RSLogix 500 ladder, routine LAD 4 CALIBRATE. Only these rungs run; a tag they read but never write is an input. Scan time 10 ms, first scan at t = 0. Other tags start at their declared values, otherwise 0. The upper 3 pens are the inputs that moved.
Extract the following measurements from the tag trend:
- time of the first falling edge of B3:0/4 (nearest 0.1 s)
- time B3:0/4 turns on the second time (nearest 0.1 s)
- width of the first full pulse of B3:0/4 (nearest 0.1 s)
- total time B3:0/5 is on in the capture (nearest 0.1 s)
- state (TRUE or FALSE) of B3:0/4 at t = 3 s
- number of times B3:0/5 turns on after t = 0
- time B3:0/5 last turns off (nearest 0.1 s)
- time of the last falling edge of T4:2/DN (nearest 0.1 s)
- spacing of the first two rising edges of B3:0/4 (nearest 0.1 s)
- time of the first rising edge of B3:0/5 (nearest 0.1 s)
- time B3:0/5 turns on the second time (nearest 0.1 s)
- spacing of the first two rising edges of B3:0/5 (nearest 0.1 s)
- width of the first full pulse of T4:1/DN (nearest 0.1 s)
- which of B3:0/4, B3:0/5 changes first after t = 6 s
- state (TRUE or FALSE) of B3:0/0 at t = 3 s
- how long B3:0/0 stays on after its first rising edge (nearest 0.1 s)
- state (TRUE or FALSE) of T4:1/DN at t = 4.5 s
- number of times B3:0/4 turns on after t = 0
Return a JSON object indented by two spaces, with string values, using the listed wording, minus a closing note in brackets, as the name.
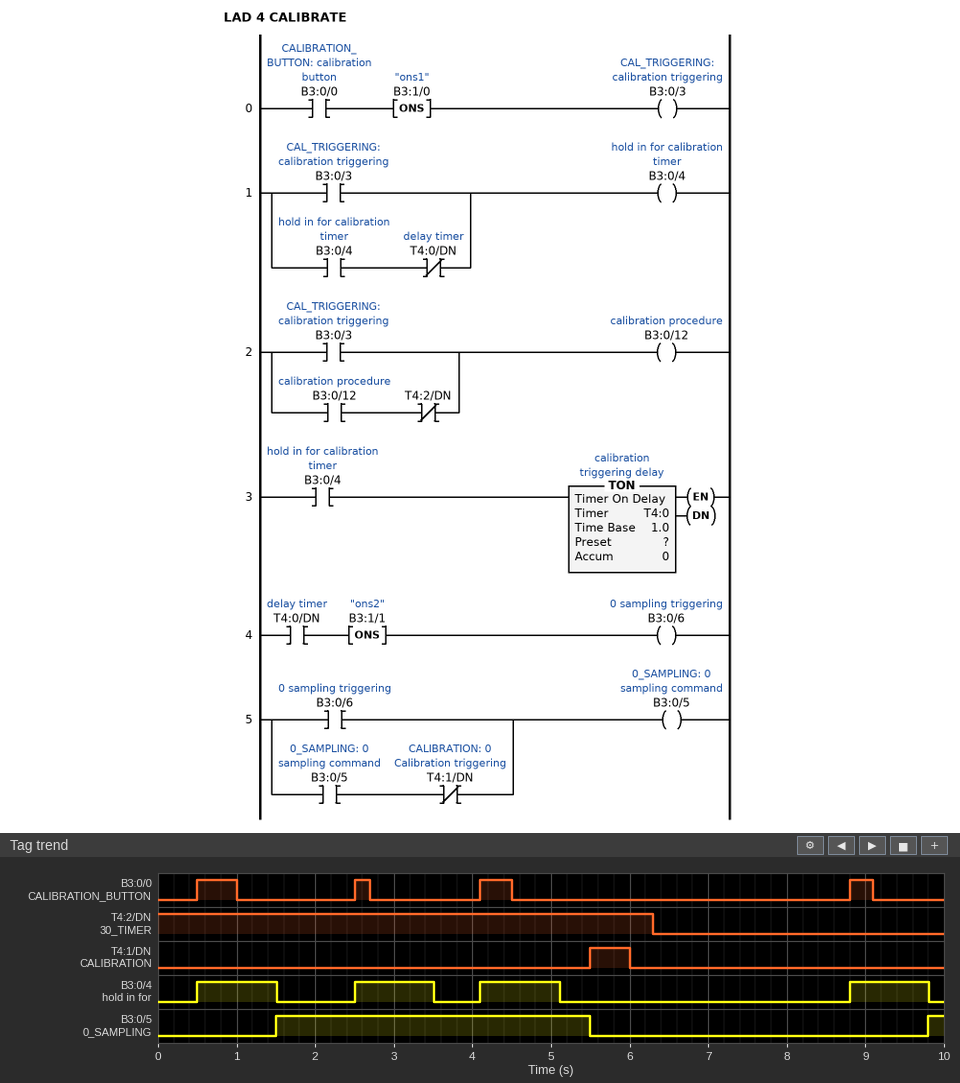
{
  "time of the first falling edge of B3:0/4": "1.5 s",
  "time B3:0/4 turns on the second time": "2.5 s",
  "width of the first full pulse of B3:0/4": "1.0 s",
  "total time B3:0/5 is on in the capture": "4.2 s",
  "state (TRUE or FALSE) of B3:0/4 at t = 3 s": "TRUE",
  "number of times B3:0/5 turns on after t = 0": "2",
  "time B3:0/5 last turns off": "5.5 s",
  "time of the last falling edge of T4:2/DN": "6.3 s",
  "spacing of the first two rising edges of B3:0/4": "2.0 s",
  "time of the first rising edge of B3:0/5": "1.5 s",
  "time B3:0/5 turns on the second time": "9.8 s",
  "spacing of the first two rising edges of B3:0/5": "8.3 s",
  "width of the first full pulse of T4:1/DN": "0.5 s",
  "which of B3:0/4, B3:0/5 changes first after t = 6 s": "B3:0/4",
  "state (TRUE or FALSE) of B3:0/0 at t = 3 s": "FALSE",
  "how long B3:0/0 stays on after its first rising edge": "0.5 s",
  "state (TRUE or FALSE) of T4:1/DN at t = 4.5 s": "FALSE",
  "number of times B3:0/4 turns on after t = 0": "4"
}
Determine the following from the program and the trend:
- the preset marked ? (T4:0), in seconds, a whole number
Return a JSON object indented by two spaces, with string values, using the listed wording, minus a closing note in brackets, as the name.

{
  "the preset marked ? (T4:0), in seconds, a whole number": "1 s"
}
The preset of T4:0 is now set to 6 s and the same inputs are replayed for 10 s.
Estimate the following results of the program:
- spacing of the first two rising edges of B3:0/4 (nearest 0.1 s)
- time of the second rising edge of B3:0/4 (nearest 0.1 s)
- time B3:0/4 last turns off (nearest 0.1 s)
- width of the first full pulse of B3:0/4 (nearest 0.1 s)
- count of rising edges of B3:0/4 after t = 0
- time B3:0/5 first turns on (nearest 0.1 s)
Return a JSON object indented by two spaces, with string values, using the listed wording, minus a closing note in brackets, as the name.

{
  "spacing of the first two rising edges of B3:0/4": "8.3 s",
  "time of the second rising edge of B3:0/4": "8.8 s",
  "time B3:0/4 last turns off": "6.5 s",
  "width of the first full pulse of B3:0/4": "6.0 s",
  "count of rising edges of B3:0/4 after t = 0": "2",
  "time B3:0/5 first turns on": "6.5 s"
}
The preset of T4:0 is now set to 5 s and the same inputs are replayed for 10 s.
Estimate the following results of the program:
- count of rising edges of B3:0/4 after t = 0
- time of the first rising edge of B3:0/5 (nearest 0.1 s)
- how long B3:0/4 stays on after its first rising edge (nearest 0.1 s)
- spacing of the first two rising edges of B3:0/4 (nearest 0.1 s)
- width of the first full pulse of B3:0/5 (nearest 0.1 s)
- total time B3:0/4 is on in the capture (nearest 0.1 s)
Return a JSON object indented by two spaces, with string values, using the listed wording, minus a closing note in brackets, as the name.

{
  "count of rising edges of B3:0/4 after t = 0": "2",
  "time of the first rising edge of B3:0/5": "5.5 s",
  "how long B3:0/4 stays on after its first rising edge": "5.0 s",
  "spacing of the first two rising edges of B3:0/4": "8.3 s",
  "width of the first full pulse of B3:0/5": "0.0 s",
  "total time B3:0/4 is on in the capture": "6.2 s"
}
